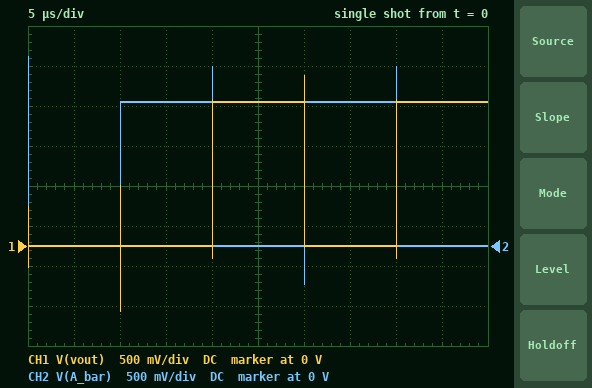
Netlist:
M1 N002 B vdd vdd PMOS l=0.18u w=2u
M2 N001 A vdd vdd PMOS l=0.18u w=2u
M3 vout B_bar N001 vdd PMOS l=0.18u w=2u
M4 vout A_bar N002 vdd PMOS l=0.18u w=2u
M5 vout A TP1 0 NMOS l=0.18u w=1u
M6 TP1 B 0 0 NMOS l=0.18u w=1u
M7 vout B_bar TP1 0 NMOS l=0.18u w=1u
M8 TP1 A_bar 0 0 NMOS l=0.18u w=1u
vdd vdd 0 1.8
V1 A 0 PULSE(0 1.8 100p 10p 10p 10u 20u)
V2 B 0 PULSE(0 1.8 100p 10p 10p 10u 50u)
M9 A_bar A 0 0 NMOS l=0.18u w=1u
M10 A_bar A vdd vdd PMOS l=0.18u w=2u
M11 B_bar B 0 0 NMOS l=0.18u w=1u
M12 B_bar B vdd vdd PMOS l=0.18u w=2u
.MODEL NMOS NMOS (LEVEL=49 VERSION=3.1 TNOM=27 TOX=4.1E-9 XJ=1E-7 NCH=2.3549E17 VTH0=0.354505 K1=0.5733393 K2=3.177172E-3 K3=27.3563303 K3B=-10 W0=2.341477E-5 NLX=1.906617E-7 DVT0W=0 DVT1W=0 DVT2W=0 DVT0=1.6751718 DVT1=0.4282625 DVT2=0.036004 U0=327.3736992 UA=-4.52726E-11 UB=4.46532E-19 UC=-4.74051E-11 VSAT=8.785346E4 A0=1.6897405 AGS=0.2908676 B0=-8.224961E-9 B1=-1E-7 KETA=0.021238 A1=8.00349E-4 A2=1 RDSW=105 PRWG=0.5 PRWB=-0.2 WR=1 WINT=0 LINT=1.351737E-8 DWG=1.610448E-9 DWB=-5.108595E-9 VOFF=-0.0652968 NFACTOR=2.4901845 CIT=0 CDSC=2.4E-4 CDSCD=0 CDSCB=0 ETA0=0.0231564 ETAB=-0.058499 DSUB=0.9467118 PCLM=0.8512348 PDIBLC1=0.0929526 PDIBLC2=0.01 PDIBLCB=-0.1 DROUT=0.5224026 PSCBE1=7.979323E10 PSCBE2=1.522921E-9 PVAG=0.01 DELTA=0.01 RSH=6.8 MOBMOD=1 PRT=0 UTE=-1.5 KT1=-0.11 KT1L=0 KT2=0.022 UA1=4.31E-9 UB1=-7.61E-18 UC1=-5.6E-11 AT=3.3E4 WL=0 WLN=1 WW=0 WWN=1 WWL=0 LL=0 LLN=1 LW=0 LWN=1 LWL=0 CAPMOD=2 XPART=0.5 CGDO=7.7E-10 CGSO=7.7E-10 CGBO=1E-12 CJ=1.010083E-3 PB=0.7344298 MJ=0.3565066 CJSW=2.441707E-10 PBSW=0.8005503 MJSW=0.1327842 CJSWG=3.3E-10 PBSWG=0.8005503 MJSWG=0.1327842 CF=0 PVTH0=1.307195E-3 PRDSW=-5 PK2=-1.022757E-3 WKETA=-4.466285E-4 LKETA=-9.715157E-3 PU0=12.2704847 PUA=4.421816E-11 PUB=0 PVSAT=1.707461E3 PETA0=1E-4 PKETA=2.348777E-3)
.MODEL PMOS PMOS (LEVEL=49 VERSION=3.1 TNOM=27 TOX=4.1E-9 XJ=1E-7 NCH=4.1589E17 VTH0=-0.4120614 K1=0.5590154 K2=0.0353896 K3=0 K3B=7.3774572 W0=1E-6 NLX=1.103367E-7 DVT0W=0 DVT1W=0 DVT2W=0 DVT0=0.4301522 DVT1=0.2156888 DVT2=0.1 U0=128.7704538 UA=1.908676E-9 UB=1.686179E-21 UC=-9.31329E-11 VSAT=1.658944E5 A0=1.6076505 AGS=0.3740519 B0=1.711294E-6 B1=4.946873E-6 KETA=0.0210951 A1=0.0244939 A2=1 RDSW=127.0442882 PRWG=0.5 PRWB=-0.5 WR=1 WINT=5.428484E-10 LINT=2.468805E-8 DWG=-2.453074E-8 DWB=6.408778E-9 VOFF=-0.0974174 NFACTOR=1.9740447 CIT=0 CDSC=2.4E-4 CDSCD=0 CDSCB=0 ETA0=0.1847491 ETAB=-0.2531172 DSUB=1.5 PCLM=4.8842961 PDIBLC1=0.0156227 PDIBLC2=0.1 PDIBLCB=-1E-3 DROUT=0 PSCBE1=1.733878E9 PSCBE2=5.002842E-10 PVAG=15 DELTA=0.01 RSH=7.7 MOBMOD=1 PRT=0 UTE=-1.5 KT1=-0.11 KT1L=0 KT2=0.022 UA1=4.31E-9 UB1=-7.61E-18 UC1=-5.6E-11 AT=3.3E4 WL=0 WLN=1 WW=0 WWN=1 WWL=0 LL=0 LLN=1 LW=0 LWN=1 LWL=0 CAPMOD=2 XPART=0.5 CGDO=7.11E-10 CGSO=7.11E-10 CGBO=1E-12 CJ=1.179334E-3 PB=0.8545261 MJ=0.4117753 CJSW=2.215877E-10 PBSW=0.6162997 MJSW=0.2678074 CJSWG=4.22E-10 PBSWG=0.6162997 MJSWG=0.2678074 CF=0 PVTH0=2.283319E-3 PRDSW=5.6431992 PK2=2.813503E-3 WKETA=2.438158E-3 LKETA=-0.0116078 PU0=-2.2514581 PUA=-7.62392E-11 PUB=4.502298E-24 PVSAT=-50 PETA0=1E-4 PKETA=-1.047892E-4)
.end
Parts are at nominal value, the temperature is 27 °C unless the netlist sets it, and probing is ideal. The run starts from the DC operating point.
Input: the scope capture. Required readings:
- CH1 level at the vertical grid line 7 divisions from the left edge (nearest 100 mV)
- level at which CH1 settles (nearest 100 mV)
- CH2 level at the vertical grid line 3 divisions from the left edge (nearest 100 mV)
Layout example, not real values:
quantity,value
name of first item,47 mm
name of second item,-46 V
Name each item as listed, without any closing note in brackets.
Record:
quantity,value
CH1 level at the vertical grid line 7 divisions from the left edge,0 V
level at which CH1 settles,1.8 V
CH2 level at the vertical grid line 3 divisions from the left edge,1.8 V
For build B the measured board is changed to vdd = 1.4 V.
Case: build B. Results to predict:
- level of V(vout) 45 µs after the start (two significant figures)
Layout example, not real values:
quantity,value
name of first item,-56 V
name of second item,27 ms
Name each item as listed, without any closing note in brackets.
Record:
quantity,value
level of V(vout) 45 µs after the start,1.4 V
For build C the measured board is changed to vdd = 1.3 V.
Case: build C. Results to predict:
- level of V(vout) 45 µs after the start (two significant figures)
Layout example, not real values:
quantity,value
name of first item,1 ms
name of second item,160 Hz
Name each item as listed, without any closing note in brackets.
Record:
quantity,value
level of V(vout) 45 µs after the start,1.3 V
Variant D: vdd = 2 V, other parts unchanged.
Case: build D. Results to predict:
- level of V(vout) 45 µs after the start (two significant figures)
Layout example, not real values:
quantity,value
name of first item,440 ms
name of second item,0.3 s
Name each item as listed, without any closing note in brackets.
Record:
quantity,value
level of V(vout) 45 µs after the start,2.0 V
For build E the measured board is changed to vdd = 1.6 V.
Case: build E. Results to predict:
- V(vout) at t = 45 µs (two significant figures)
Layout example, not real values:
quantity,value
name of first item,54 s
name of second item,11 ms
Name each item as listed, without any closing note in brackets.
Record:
quantity,value
V(vout) at t = 45 µs,1.6 V
